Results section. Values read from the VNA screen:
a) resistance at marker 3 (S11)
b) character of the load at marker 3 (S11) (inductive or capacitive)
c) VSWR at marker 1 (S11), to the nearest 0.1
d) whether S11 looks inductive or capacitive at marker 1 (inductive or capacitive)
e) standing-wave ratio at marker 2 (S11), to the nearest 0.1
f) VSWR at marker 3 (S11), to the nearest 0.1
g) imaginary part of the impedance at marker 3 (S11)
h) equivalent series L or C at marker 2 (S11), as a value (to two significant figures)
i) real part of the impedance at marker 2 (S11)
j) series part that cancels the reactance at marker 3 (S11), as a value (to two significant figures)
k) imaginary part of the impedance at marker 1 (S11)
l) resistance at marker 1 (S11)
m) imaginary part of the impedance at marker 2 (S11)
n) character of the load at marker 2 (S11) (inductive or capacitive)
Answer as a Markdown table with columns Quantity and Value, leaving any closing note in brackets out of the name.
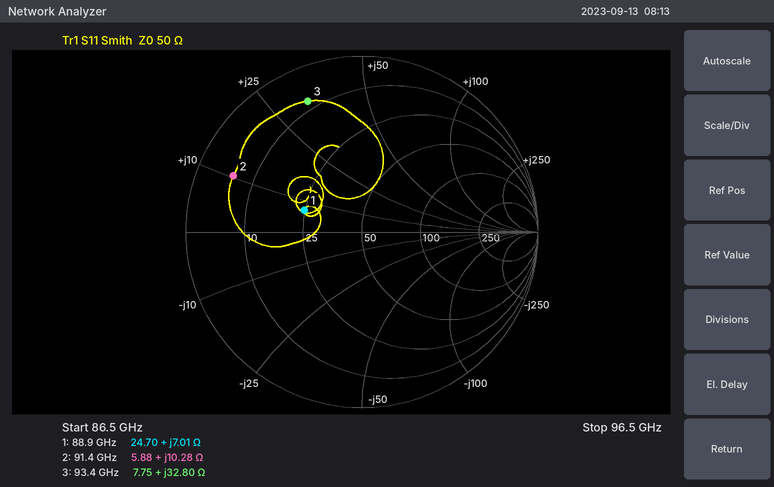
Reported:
| Quantity | Value |
|---|---|
| resistance at marker 3 | 7.75 Ω |
| character of the load at marker 3 (S11) | inductive |
| VSWR at marker 1 (S11), to the nearest 0.1 | 2.1 |
| whether S11 looks inductive or capacitive at marker 1 | inductive |
| standing-wave ratio at marker 2 (S11), to the nearest 0.1 | 8.9 |
| VSWR at marker 3 (S11), to the nearest 0.1 | 9.3 |
| imaginary part of the impedance at marker 3 | +32.80 Ω |
| equivalent series L or C at marker 2 (S11), as a value | 18 pH |
| real part of the impedance at marker 2 | 5.88 Ω |
| series part that cancels the reactance at marker 3 (S11), as a value | 52 fF |
| imaginary part of the impedance at marker 1 | +7.01 Ω |
| resistance at marker 1 | 24.70 Ω |
| imaginary part of the impedance at marker 2 | +10.28 Ω |
| character of the load at marker 2 (S11) | inductive |
